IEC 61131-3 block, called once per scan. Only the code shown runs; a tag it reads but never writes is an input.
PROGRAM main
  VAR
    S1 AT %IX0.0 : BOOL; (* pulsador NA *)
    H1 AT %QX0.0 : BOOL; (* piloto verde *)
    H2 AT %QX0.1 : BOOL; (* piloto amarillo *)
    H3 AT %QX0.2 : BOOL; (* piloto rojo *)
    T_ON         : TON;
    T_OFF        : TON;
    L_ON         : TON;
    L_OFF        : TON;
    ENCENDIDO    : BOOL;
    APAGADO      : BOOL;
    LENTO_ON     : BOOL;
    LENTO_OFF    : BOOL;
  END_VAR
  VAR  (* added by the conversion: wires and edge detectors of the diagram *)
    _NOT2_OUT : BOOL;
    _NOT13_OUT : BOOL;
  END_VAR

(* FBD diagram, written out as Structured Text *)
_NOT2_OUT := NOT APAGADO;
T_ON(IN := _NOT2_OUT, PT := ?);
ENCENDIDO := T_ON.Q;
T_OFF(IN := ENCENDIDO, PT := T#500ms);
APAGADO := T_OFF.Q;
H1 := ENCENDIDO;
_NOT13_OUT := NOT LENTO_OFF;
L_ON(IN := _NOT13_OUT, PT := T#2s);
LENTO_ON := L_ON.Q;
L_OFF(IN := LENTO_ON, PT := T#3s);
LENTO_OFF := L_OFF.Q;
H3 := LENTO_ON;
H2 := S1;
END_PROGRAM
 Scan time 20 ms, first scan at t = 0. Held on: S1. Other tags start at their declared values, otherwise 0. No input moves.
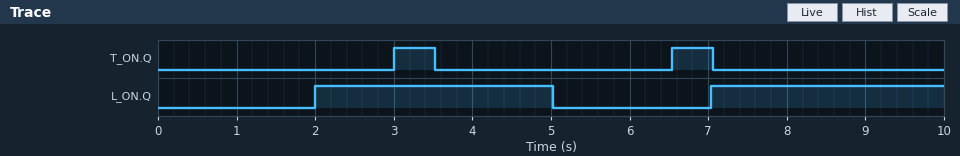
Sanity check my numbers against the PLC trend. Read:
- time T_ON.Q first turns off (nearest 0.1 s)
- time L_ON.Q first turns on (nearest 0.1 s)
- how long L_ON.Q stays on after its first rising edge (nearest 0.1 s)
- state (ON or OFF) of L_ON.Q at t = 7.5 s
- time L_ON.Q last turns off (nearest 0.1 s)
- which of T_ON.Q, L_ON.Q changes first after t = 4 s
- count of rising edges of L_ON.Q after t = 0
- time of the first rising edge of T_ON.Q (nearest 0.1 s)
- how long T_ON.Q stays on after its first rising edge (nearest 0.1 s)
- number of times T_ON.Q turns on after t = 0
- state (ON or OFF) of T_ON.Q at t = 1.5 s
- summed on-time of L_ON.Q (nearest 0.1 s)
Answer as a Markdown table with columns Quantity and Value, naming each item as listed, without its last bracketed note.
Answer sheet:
| Quantity | Value |
|---|---|
| time T_ON.Q first turns off | 3.5 s |
| time L_ON.Q first turns on | 2.0 s |
| how long L_ON.Q stays on after its first rising edge | 3.0 s |
| state (ON or OFF) of L_ON.Q at t = 7.5 s | ON |
| time L_ON.Q last turns off | 5.0 s |
| which of T_ON.Q, L_ON.Q changes first after t = 4 s | L_ON.Q |
| count of rising edges of L_ON.Q after t = 0 | 2 |
| time of the first rising edge of T_ON.Q | 3.0 s |
| how long T_ON.Q stays on after its first rising edge | 0.5 s |
| number of times T_ON.Q turns on after t = 0 | 2 |
| state (ON or OFF) of T_ON.Q at t = 1.5 s | OFF |
| summed on-time of L_ON.Q | 6.0 s |
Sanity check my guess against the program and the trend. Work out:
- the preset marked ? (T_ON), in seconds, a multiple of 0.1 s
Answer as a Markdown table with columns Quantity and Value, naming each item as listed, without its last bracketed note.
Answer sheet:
| Quantity | Value |
|---|---|
| the preset marked ? (T_ON), in seconds, a multiple of 0.1 s | 3.0 s |
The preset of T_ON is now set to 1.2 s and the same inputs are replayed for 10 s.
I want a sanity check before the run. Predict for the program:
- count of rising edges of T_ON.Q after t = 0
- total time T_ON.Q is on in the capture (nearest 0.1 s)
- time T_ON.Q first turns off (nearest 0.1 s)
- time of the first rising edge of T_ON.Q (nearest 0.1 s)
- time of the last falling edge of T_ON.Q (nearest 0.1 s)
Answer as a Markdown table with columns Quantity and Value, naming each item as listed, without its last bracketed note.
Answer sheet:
| Quantity | Value |
|---|---|
| count of rising edges of T_ON.Q after t = 0 | 6 |
| total time T_ON.Q is on in the capture | 2.7 s |
| time T_ON.Q first turns off | 1.7 s |
| time of the first rising edge of T_ON.Q | 1.2 s |
| time of the last falling edge of T_ON.Q | 8.7 s |
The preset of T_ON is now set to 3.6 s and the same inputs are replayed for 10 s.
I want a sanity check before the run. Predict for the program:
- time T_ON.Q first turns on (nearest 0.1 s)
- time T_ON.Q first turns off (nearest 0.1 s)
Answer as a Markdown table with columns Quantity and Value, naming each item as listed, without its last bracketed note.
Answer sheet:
| Quantity | Value |
|---|---|
| time T_ON.Q first turns on | 3.6 s |
| time T_ON.Q first turns off | 4.1 s |
